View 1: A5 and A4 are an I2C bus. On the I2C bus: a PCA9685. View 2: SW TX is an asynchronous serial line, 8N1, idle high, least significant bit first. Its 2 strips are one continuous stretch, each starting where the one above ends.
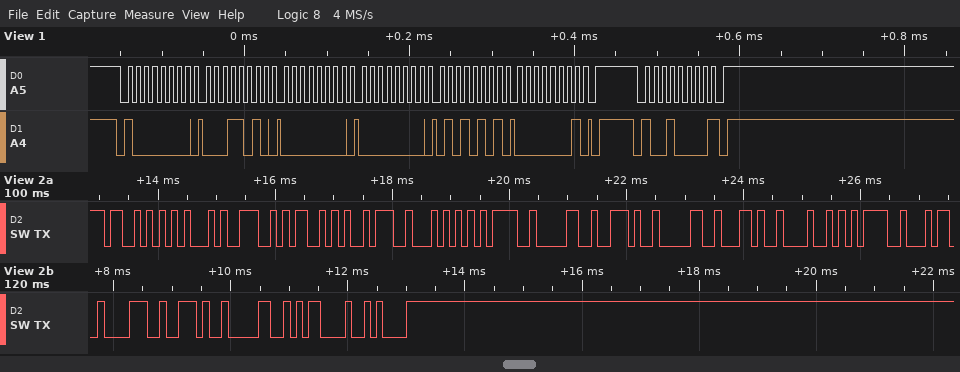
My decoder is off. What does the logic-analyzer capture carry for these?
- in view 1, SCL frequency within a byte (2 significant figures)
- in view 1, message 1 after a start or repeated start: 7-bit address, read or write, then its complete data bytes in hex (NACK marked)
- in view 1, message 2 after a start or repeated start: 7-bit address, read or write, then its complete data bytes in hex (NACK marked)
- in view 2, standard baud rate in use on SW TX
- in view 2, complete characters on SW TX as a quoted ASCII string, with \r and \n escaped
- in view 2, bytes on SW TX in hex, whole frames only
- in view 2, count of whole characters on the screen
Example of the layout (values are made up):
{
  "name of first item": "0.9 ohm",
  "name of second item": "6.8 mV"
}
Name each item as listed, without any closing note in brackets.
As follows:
{
  "in view 1, SCL frequency within a byte": "100 kHz",
  "in view 1, message 1 after a start or repeated start: 7-bit address, read or write, then its complete data bytes in hex": "0x40 write: 1A 00 00 55 01",
  "in view 1, message 2 after a start or repeated start: 7-bit address, read or write, then its complete data bytes in hex": "0x48 write NACK",
  "in view 2, standard baud rate in use on SW TX": "9600 baud",
  "in view 2, complete characters on SW TX as a quoted ASCII string, with \\r and \\n escaped": "\"SENS:T=0.0,H=48.0\\r\\n\"",
  "in view 2, bytes on SW TX in hex, whole frames only": "53 45 4E 53 3A 54 3D 30 2E 30 2C 48 3D 34 38 2E 30 0D 0A",
  "in view 2, count of whole characters on the screen": "19"
}
